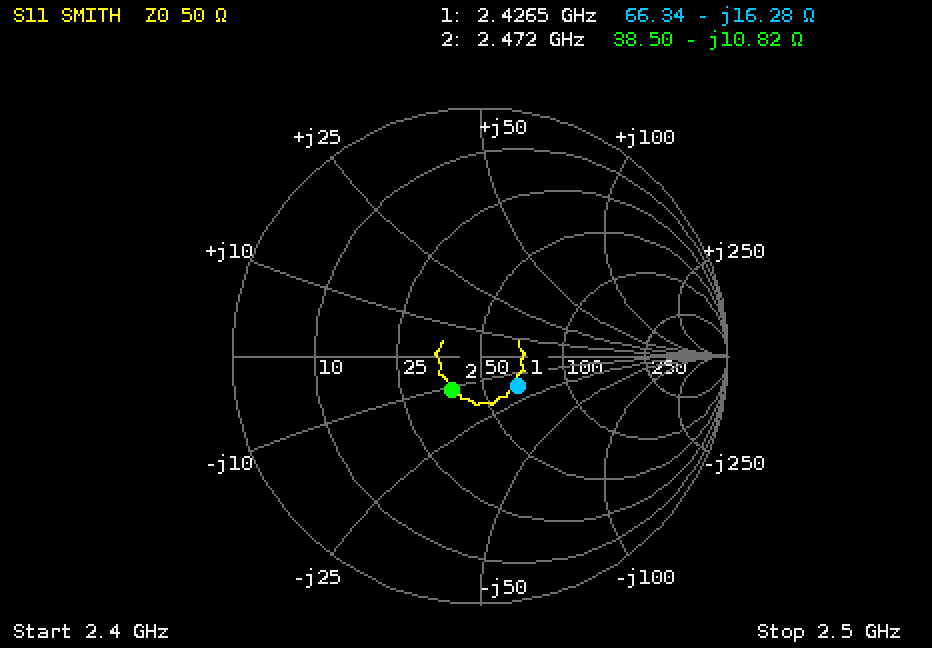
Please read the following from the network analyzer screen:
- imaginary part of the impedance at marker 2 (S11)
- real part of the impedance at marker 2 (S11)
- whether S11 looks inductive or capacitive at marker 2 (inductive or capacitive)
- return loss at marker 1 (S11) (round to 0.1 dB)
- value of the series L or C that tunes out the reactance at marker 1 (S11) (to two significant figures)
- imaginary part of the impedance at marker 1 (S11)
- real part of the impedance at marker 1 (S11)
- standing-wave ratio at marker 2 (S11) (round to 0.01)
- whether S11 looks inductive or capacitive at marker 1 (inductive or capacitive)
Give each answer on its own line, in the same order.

-10.82 Ω
38.50 Ω
capacitive
14.1 dB
1.1 nH
-16.28 Ω
66.34 Ω
1.43
capacitive
